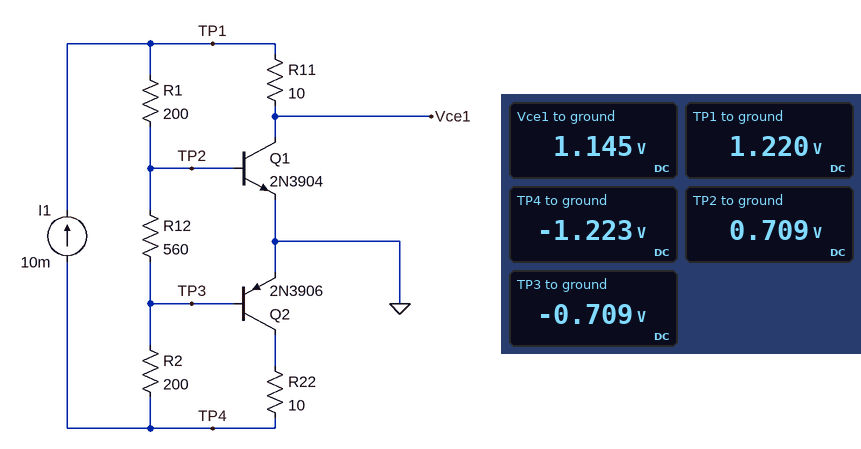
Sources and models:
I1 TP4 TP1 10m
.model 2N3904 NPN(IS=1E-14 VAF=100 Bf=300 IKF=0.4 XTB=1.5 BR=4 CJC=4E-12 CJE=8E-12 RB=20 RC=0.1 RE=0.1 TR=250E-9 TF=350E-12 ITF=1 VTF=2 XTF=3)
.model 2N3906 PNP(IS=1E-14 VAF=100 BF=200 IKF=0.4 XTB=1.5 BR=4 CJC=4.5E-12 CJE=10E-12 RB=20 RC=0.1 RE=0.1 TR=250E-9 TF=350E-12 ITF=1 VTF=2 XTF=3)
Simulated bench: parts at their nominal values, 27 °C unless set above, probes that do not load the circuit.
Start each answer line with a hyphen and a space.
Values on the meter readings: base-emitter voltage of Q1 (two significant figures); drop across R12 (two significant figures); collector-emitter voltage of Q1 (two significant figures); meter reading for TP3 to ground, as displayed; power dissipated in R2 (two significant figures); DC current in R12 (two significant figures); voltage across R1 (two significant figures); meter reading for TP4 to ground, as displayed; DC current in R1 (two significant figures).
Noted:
- 710 mV
- 1.4 V
- 1.1 V
- -0.709 V
- 1.3 mW
- 2.5 mA
- 510 mV
- -1.223 V
- 2.6 mA
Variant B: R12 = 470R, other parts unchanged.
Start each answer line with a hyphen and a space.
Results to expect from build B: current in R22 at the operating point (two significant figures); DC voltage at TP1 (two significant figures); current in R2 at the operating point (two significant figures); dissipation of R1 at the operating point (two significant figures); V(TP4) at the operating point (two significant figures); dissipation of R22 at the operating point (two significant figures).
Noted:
- 7.0 mA
- 1.3 V
- 3.0 mA
- 1.8 mW
- -1.3 V
- 480 µW
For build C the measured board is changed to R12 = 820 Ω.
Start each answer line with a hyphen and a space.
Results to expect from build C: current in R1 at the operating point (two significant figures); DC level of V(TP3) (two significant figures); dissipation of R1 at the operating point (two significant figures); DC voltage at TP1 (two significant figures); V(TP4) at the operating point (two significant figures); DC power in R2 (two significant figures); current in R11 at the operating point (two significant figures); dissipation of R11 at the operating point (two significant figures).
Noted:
- 1.8 mA
- -710 mV
- 620 µW
- 1.1 V
- -1.1 V
- 630 µW
- 8.2 mA
- 680 µW
